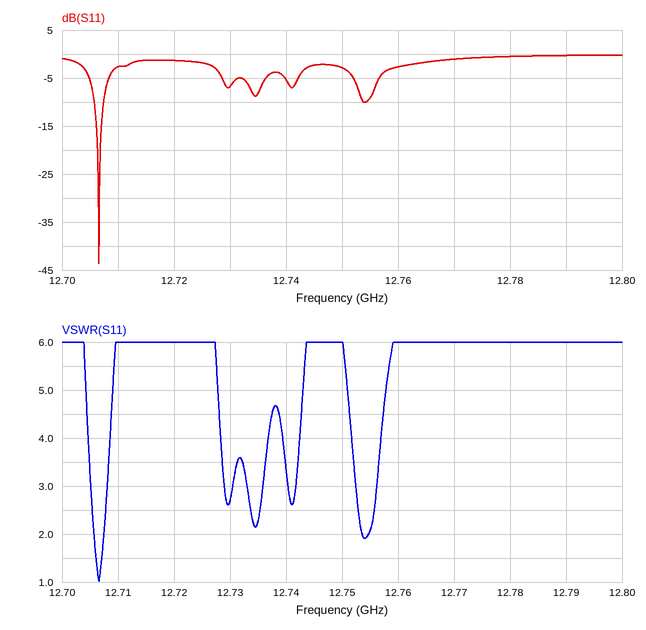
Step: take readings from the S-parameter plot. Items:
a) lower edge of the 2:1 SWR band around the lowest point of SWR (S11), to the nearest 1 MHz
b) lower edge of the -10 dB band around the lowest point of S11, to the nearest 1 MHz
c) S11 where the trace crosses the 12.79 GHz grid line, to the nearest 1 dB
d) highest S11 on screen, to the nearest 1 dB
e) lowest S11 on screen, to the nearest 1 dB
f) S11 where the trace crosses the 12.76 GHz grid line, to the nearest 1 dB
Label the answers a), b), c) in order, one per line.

a) 12.706 GHz
b) 12.706 GHz
c) 0 dB
d) 0 dB
e) -44 dB
f) -3 dB
